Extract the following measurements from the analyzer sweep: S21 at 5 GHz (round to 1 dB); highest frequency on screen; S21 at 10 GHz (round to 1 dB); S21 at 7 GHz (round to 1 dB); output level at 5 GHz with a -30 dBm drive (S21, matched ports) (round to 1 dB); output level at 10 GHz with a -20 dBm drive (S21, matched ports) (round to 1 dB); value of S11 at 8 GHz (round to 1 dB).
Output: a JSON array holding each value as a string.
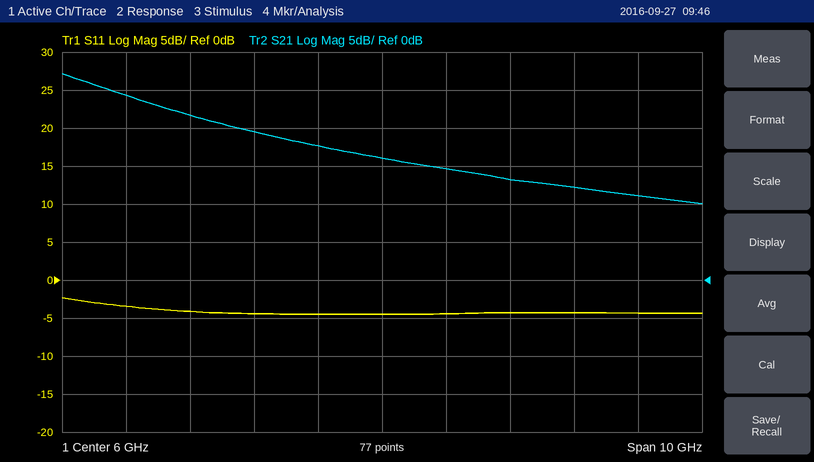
["18 dB", "11 GHz", "11 dB", "15 dB", "-12 dBm", "-9 dBm", "-4 dB"]
